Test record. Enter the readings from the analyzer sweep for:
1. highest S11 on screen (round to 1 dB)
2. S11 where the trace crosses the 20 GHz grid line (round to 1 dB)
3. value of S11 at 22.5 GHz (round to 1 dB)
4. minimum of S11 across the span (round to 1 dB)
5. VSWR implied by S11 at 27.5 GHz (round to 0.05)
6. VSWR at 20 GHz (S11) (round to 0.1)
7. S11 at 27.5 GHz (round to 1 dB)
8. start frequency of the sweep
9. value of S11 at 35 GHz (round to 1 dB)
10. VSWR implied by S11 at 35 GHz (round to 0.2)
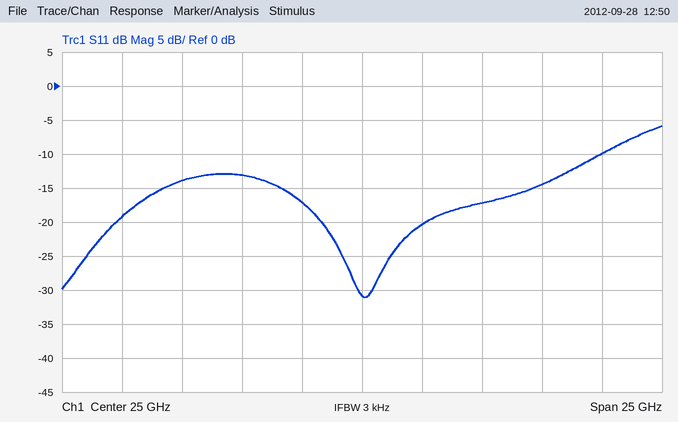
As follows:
-6 dB
-13 dB
-17 dB
-31 dB
1.20
1.6
-20 dB
12.5 GHz
-10 dB
2.0
